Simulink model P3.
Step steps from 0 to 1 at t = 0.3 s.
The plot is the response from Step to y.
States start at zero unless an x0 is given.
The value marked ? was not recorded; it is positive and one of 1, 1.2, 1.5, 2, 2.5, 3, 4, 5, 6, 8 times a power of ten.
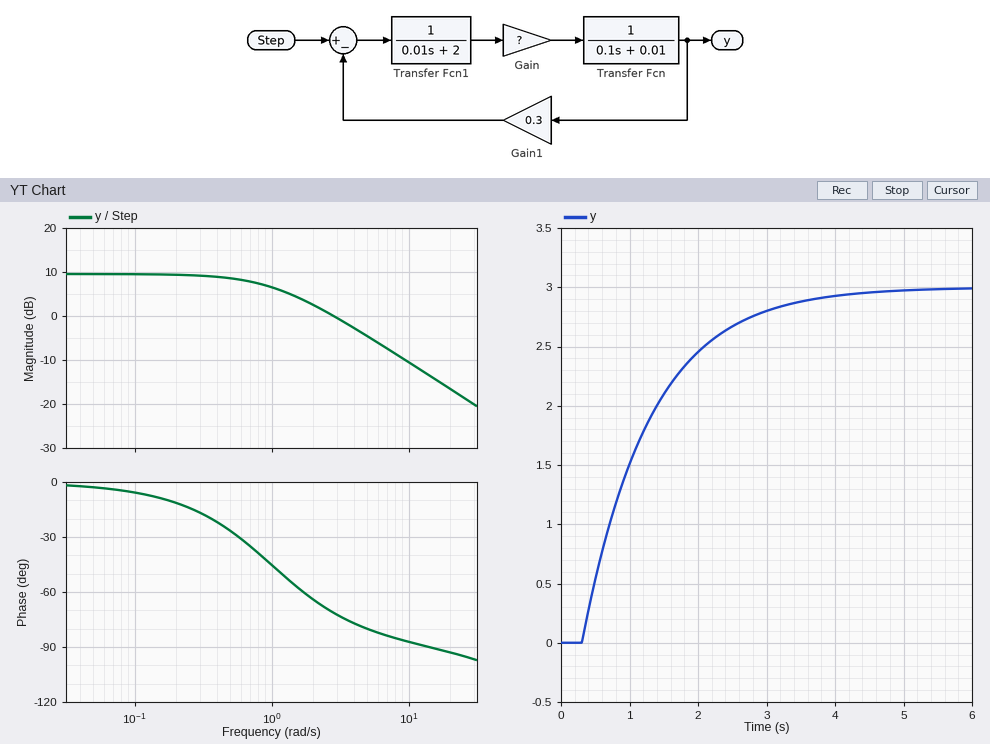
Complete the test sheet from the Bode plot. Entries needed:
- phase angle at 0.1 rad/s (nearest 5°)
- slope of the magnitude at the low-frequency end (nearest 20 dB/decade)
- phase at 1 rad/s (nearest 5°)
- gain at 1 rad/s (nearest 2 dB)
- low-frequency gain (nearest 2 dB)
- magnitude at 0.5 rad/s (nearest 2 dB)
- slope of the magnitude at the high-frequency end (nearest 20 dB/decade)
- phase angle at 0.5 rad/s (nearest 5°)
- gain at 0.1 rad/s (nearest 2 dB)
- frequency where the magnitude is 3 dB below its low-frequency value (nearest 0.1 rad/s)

-5°
0 dB/decade
-45°
6 dB
10 dB
8 dB
-20 dB/decade
-25°
10 dB
1.0 rad/s
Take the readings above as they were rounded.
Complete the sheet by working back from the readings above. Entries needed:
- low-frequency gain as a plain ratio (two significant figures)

3.2
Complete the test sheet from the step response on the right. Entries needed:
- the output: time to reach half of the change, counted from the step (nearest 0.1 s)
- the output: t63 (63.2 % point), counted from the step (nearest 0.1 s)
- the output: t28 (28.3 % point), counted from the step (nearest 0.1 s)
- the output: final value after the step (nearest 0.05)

0.7 s
1.0 s
0.3 s
3.00
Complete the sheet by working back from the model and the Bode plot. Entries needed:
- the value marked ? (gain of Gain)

0.6
